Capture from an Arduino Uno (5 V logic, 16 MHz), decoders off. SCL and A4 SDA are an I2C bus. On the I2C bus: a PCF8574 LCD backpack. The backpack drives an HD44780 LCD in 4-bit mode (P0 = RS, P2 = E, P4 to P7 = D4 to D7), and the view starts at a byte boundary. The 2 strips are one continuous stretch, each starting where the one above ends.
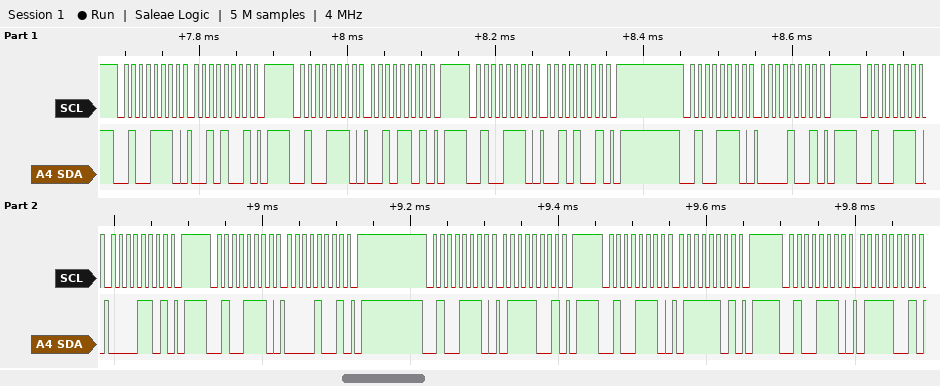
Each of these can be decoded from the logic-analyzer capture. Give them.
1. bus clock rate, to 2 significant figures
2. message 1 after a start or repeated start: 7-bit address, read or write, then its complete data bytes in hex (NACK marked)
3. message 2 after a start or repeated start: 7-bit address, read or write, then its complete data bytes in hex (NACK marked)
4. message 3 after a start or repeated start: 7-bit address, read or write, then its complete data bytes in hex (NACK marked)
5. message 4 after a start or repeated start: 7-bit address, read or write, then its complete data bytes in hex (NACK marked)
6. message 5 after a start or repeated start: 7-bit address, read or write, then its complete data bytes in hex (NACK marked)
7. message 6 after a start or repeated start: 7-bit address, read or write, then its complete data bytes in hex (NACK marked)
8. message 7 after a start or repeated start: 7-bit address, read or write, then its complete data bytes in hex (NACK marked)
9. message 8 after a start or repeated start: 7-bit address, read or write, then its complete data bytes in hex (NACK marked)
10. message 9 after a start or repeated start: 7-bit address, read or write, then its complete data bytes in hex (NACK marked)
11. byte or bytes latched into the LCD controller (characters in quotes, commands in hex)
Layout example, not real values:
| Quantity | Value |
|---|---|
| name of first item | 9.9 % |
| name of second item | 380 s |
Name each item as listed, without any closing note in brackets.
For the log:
| Quantity | Value |
|---|---|
| bus clock rate, to 2 significant figures | 100 kHz |
| message 1 after a start or repeated start: 7-bit address, read or write, then its complete data bytes in hex | 0x27 write: 29 |
| message 2 after a start or repeated start: 7-bit address, read or write, then its complete data bytes in hex | 0x27 write: 2D |
| message 3 after a start or repeated start: 7-bit address, read or write, then its complete data bytes in hex | 0x27 write: 29 |
| message 4 after a start or repeated start: 7-bit address, read or write, then its complete data bytes in hex | 0x27 write: 09 |
| message 5 after a start or repeated start: 7-bit address, read or write, then its complete data bytes in hex | 0x27 write: 0D |
| message 6 after a start or repeated start: 7-bit address, read or write, then its complete data bytes in hex | 0x27 write: 09 |
| message 7 after a start or repeated start: 7-bit address, read or write, then its complete data bytes in hex | 0x27 write: 79 |
| message 8 after a start or repeated start: 7-bit address, read or write, then its complete data bytes in hex | 0x27 write: 7D |
| message 9 after a start or repeated start: 7-bit address, read or write, then its complete data bytes in hex | 0x27 write: 79 |
| byte or bytes latched into the LCD controller | ' ' |
